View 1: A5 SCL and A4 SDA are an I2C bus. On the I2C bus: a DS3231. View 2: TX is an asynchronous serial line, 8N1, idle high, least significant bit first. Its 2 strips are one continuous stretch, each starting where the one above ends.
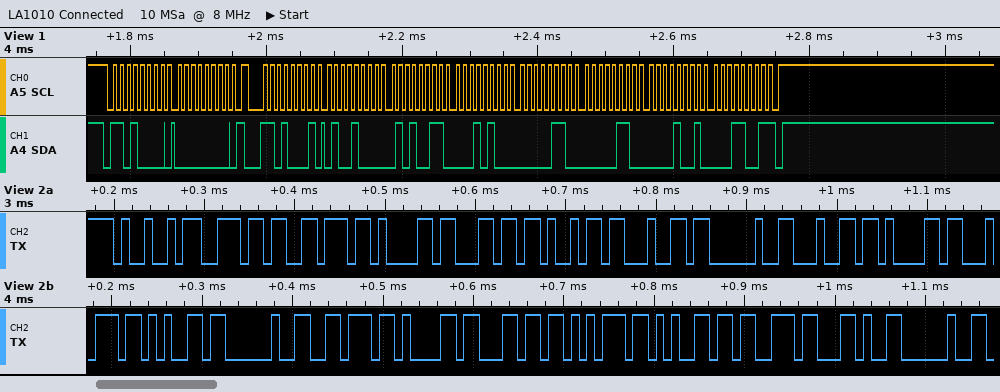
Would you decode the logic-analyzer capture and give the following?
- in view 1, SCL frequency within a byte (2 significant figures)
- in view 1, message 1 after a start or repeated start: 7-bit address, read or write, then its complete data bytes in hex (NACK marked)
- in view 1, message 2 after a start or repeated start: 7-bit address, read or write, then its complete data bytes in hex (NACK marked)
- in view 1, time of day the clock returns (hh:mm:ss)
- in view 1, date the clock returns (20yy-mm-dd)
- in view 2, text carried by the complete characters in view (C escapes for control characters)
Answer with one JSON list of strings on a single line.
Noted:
["100 kHz", "0x68 write: 00", "0x68 read: 48 53 14 06 06 09 19 NACK", "14:53:48", "2019-09-06", "\"Invalid date values, \""]
